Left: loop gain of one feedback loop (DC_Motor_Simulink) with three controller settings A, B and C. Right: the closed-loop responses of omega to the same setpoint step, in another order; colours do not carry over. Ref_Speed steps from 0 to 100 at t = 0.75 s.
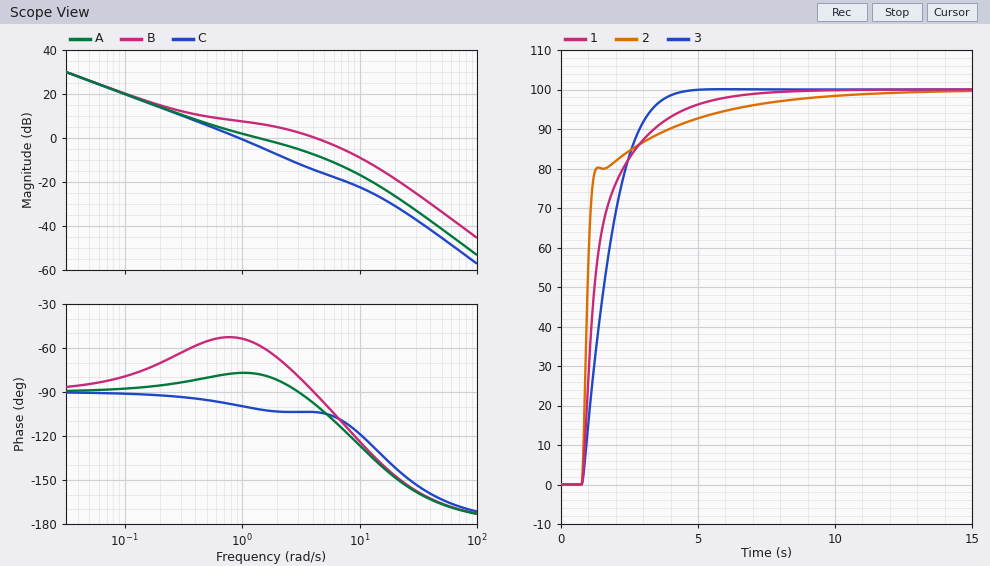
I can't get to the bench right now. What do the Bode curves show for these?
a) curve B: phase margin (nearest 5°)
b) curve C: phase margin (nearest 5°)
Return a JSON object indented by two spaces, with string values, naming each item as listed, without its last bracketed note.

{
  "curve B: phase margin": "90°",
  "curve C: phase margin": "80°"
}
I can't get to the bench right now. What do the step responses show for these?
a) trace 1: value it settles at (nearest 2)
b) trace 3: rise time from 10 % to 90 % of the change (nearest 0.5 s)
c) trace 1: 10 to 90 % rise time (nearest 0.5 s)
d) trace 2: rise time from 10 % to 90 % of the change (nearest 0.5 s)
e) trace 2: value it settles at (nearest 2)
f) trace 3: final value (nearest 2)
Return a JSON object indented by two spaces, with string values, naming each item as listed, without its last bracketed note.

{
  "trace 1: value it settles at": "100",
  "trace 3: rise time from 10 % to 90 % of the change": "2.0 s",
  "trace 1: 10 to 90 % rise time": "2.5 s",
  "trace 2: rise time from 10 % to 90 % of the change": "3.0 s",
  "trace 2: value it settles at": "100",
  "trace 3: final value": "100"
}
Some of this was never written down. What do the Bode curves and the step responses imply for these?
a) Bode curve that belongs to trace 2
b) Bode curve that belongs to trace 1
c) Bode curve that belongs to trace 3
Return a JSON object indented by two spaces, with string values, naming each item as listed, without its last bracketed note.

{
  "Bode curve that belongs to trace 2": "B",
  "Bode curve that belongs to trace 1": "A",
  "Bode curve that belongs to trace 3": "C"
}
